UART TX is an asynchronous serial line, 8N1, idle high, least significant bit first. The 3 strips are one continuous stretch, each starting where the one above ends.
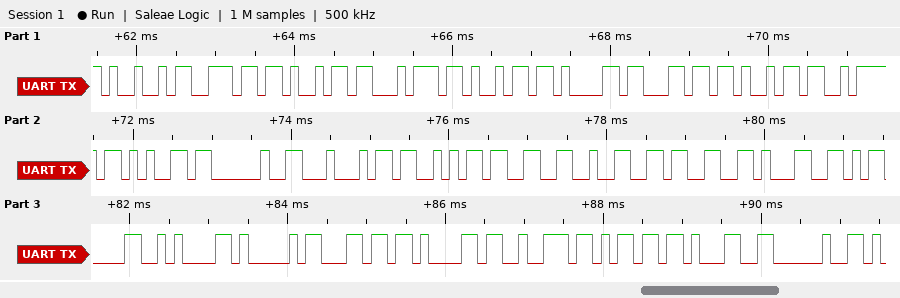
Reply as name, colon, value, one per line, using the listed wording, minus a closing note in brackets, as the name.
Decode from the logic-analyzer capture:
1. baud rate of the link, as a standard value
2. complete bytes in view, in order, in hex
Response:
baud rate of the link, as a standard value: 9600 baud
complete bytes in view, in order, in hex: 49 6E 69 74 69 61 6C 69 7A 65 20 44 53 33 32 33 31 0D 0A 41 6C 61 72 6D 31 20
